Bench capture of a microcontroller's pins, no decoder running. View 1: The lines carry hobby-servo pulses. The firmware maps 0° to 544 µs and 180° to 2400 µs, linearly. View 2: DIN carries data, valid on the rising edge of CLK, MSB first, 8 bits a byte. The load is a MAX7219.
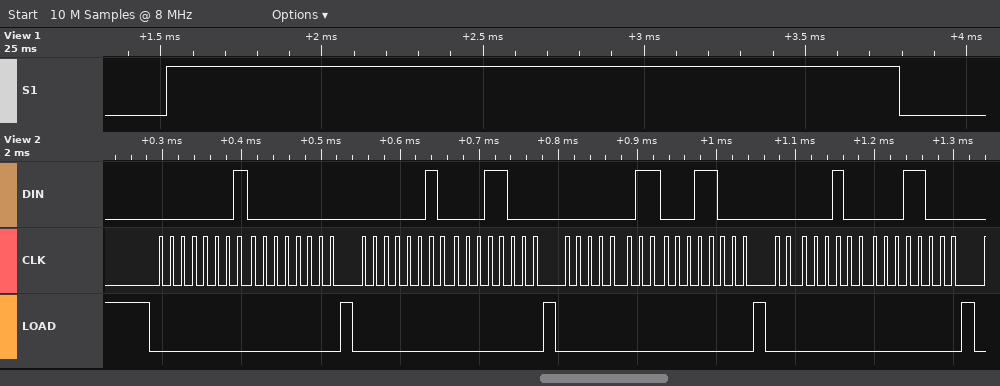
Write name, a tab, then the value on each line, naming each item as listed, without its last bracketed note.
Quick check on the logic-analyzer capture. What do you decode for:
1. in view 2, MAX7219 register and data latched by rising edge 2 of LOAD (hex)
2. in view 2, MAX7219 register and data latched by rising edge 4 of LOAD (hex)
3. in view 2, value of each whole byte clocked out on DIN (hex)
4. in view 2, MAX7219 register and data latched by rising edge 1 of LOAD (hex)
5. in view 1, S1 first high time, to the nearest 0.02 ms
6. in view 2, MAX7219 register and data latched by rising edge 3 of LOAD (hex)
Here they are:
in view 2, MAX7219 register and data latched by rising edge 2 of LOAD	register 0x2, data 0x18
in view 2, MAX7219 register and data latched by rising edge 4 of LOAD	register 0x4, data 0x18
in view 2, value of each whole byte clocked out on DIN	01 00 02 18 03 18 04 18
in view 2, MAX7219 register and data latched by rising edge 1 of LOAD	register 0x1, data 0x00
in view 1, S1 first high time, to the nearest 0.02 ms	2.28 ms
in view 2, MAX7219 register and data latched by rising edge 3 of LOAD	register 0x3, data 0x18
